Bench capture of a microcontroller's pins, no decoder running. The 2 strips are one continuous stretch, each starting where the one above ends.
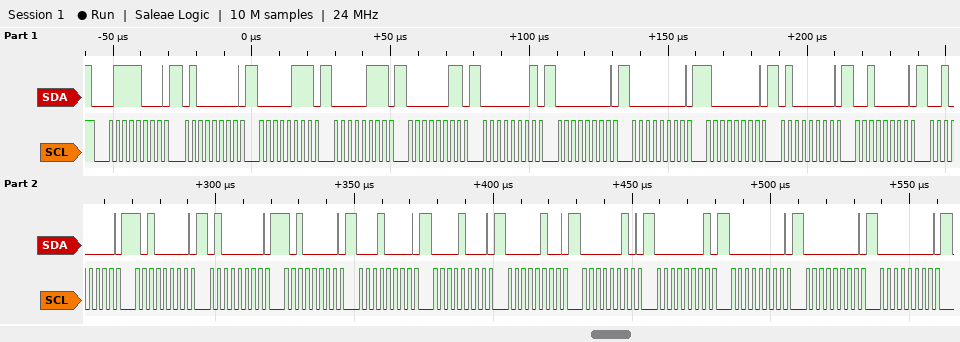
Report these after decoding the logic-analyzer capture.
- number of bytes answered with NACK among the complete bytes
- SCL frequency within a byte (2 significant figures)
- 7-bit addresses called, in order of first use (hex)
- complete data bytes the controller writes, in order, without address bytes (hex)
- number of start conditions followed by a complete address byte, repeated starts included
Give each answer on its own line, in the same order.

0
400 kHz
0x3C
40 07 07 03 01 00 00 80 40 20 20 A0 40 A0 10 08 04 02 01 00 00 00
1
